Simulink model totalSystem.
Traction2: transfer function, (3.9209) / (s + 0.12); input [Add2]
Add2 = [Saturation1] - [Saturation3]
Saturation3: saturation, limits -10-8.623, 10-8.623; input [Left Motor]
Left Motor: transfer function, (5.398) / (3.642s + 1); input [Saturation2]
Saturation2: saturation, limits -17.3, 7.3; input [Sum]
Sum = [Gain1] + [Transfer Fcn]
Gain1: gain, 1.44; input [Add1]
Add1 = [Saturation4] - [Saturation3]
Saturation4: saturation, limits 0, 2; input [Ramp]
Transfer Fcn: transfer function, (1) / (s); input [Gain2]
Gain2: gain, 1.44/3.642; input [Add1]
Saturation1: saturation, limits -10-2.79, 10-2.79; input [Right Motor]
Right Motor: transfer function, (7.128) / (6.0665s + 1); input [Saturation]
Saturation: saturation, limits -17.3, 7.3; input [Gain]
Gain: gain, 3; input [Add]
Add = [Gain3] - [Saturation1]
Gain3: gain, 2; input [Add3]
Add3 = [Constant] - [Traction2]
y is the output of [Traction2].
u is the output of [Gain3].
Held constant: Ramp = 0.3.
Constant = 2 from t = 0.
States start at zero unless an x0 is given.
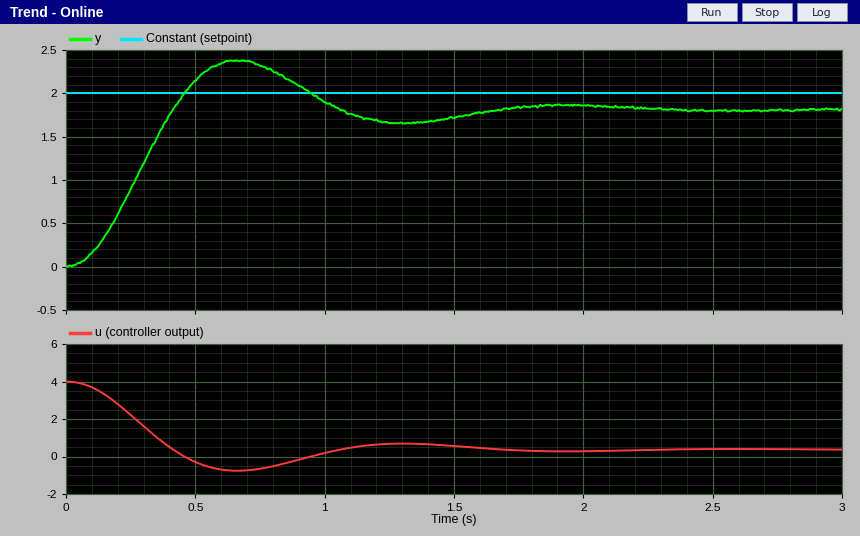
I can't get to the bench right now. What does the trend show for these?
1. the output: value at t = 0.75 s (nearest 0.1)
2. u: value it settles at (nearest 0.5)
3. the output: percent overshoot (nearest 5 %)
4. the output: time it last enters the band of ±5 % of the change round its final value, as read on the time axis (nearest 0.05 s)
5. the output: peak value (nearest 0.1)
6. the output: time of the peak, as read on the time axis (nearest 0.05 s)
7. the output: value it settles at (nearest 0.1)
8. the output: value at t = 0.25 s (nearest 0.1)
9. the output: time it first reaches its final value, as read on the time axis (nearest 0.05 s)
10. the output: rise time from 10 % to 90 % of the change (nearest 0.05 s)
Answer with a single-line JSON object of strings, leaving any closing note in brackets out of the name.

{"the output: value at t = 0.75 s": "2.3", "u: value it settles at": "0.5", "the output: percent overshoot": "30 %", "the output: time it last enters the band of ±5 % of the change round its final value, as read on the time axis": "1.50 s", "the output: peak value": "2.4", "the output: time of the peak, as read on the time axis": "0.65 s", "the output: value it settles at": "1.8", "the output: value at t = 0.25 s": "0.9", "the output: time it first reaches its final value, as read on the time axis": "0.40 s", "the output: rise time from 10 % to 90 % of the change": "0.25 s"}
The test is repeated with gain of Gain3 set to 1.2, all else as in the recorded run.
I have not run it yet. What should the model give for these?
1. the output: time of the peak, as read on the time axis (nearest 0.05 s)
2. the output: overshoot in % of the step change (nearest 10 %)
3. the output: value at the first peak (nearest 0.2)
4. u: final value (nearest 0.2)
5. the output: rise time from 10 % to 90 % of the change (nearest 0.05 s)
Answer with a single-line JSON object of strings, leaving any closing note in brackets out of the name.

{"the output: time of the peak, as read on the time axis": "0.85 s", "the output: overshoot in % of the step change": "20 %", "the output: value at the first peak": "2.0", "u: final value": "0.4", "the output: rise time from 10 % to 90 % of the change": "0.35 s"}
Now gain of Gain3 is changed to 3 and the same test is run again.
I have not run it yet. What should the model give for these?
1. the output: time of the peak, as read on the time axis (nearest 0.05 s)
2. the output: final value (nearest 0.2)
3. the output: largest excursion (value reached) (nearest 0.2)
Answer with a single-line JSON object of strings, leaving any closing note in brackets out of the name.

{"the output: time of the peak, as read on the time axis": "0.60 s", "the output: final value": "1.8", "the output: largest excursion (value reached)": "2.6"}
